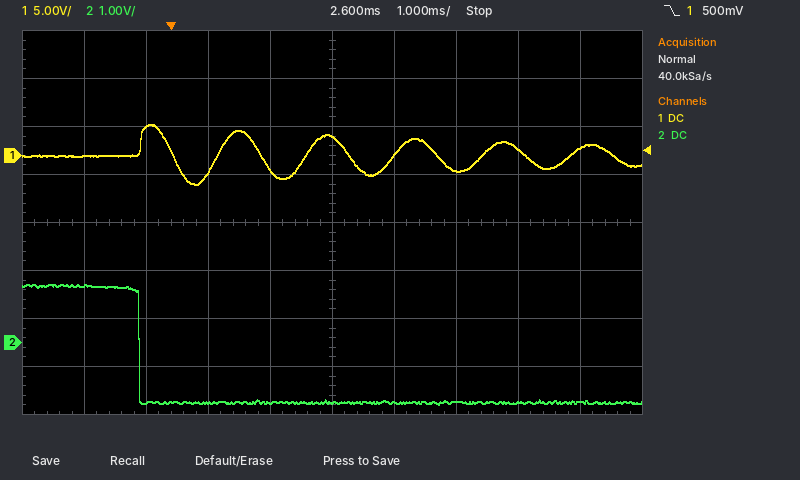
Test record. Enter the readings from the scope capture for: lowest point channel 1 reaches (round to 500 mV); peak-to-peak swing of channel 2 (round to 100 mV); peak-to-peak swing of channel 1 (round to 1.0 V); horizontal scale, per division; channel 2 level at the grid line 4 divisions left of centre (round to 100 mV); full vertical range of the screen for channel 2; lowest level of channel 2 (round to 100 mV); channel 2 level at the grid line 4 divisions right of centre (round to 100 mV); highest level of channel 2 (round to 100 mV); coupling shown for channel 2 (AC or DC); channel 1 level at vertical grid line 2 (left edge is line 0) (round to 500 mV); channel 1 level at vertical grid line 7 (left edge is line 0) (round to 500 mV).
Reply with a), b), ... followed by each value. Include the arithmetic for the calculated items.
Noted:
a) -3.0 V
b) 1.2 V − (-1.3 V) = 2.5 V
c) 6.0 V
d) 1 ms
e) 1.2 V
f) 8 V
g) -1.3 V
h) -1.2 V
i) 1.2 V
j) DC
k) 3.0 V
l) -1.5 V
